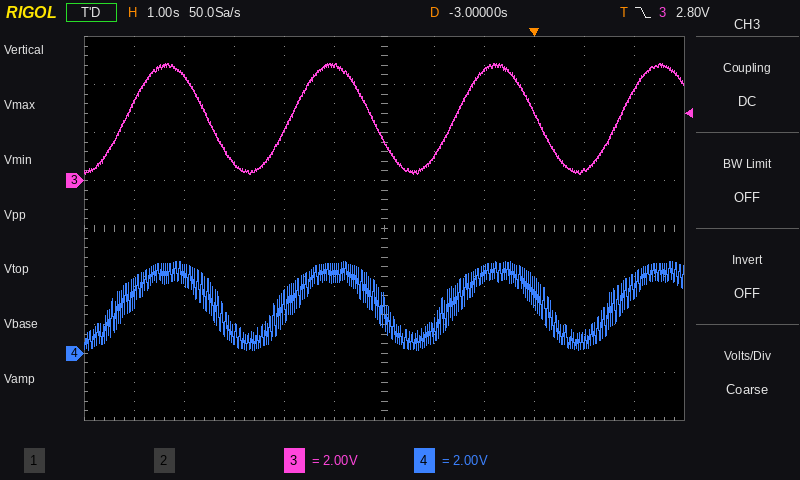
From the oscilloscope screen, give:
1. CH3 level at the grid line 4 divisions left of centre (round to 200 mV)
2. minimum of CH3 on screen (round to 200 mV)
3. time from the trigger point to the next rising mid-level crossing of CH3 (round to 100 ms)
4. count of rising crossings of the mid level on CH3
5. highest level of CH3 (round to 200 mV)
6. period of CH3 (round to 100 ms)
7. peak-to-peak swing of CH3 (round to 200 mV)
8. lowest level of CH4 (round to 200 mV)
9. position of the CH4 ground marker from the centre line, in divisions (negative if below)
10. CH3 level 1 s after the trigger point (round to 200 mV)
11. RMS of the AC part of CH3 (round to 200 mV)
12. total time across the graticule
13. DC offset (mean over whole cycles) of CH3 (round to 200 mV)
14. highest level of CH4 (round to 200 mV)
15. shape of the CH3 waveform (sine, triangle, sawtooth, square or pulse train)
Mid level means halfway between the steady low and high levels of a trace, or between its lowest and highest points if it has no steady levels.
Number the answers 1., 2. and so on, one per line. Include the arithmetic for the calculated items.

1. 4.4 V
2. 200 mV
3. 1.7 s
4. 4
5. 4.8 V
6. 3.3 s
7. 4.8 V − (200 mV) = 4.6 V
8. 200 mV
9. -2.6 div
10. 400 mV
11. 4.6 V / (2√2) ≈ 1.6 V
12. 12 s
13. (4.8 V + (200 mV)) / 2 ≈ 2.50 V, so 2.6 V to the nearest 200 mV
14. 3.8 V
15. sine
